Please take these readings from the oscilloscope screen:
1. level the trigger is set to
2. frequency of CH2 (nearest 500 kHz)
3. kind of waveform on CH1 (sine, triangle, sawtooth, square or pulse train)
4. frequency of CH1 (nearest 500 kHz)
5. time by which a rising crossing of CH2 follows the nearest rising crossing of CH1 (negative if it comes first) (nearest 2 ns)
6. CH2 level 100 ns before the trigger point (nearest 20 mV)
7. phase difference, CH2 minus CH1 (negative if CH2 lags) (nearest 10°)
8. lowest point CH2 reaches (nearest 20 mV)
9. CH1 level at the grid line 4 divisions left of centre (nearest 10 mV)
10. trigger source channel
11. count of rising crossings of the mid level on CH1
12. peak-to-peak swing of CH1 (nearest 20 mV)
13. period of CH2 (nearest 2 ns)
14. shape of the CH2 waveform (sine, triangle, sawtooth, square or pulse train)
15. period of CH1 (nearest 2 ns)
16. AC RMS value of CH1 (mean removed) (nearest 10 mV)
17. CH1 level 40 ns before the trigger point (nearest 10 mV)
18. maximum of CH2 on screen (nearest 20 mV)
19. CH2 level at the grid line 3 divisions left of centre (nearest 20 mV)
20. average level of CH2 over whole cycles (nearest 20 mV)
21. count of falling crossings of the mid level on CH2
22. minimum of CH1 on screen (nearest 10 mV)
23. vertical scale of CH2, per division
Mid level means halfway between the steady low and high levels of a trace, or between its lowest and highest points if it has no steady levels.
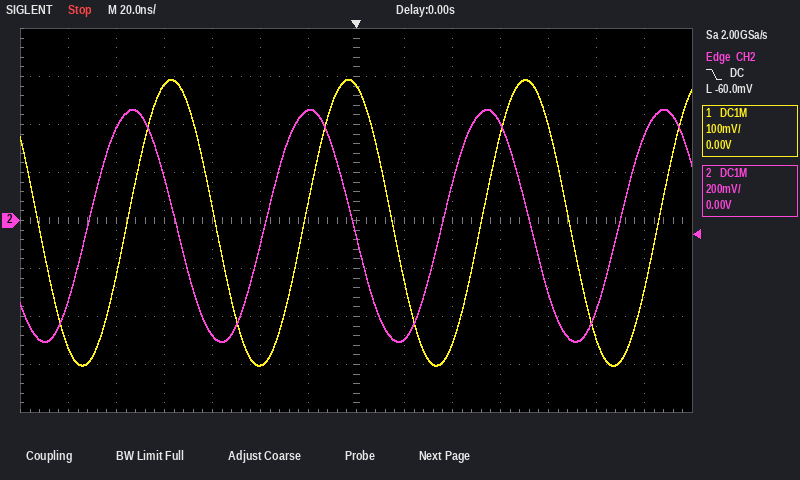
-60.0 mV
13.5 MHz
sine
13.5 MHz
-16 ns
380 mV
+80°
-500 mV
280 mV
CH2
4
600 mV
74 ns
sine
74 ns
210 mV
-300 mV
460 mV
-480 mV
-20 mV
3
-300 mV
200 mV
